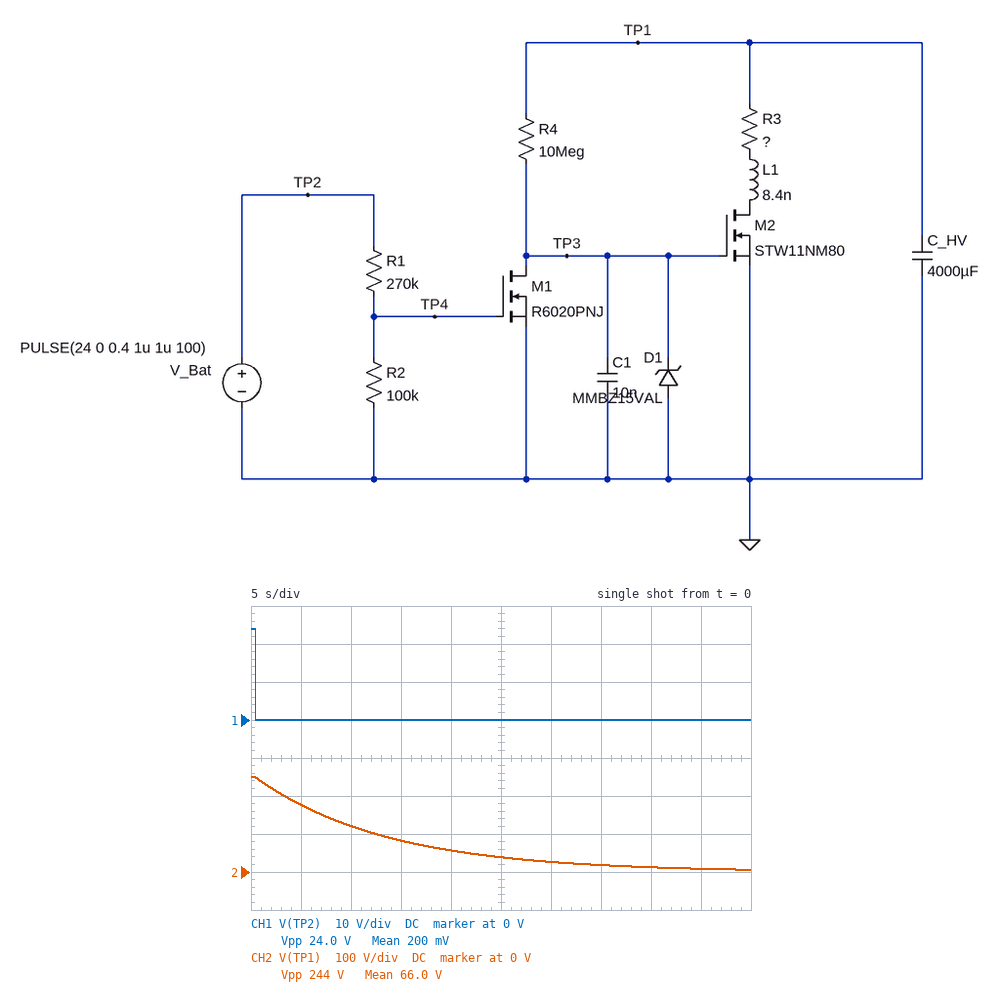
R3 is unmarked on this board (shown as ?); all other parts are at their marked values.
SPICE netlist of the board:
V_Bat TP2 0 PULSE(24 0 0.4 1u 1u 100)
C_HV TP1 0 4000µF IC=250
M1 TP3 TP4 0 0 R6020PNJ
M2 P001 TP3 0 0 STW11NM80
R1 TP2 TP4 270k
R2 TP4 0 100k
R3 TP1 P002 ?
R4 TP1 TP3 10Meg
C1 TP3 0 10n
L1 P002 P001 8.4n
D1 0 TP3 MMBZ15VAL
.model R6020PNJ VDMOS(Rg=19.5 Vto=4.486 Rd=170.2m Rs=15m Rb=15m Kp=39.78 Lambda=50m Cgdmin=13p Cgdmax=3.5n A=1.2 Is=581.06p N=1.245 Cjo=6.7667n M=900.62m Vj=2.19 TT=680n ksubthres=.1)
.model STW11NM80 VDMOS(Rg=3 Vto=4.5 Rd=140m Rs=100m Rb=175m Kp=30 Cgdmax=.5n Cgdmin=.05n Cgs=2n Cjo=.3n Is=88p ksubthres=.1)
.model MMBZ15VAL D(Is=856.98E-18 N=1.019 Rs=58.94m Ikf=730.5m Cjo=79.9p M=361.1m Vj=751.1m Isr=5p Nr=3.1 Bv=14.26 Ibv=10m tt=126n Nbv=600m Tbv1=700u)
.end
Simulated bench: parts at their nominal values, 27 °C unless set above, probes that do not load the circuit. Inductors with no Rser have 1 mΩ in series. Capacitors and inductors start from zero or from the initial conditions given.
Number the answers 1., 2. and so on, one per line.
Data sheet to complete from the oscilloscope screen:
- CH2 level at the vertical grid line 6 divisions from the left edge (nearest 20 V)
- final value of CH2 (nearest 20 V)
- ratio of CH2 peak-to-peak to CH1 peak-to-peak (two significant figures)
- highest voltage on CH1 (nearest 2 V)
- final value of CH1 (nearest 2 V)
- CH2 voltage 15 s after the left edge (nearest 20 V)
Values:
1. 20 V
2. 0 V
3. 10
4. 24 V
5. 0 V
6. 80 V
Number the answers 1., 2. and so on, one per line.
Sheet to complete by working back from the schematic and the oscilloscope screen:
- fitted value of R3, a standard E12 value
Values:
1. 3.3 kΩ
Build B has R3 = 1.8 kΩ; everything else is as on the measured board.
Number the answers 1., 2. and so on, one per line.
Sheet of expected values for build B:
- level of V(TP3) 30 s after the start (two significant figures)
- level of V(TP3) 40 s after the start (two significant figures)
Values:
1. 4.2 V
2. 4.0 V
